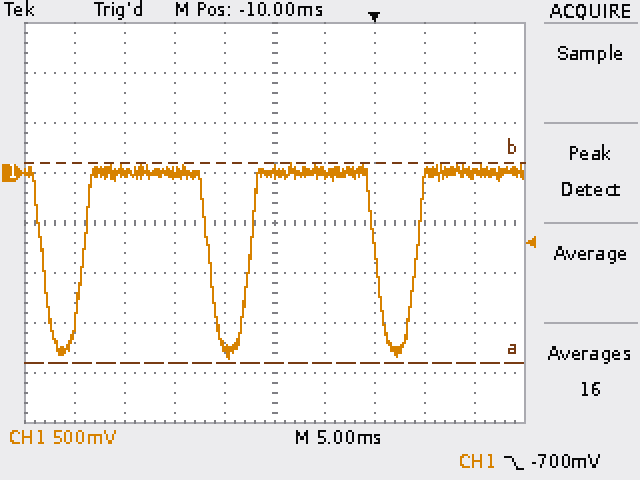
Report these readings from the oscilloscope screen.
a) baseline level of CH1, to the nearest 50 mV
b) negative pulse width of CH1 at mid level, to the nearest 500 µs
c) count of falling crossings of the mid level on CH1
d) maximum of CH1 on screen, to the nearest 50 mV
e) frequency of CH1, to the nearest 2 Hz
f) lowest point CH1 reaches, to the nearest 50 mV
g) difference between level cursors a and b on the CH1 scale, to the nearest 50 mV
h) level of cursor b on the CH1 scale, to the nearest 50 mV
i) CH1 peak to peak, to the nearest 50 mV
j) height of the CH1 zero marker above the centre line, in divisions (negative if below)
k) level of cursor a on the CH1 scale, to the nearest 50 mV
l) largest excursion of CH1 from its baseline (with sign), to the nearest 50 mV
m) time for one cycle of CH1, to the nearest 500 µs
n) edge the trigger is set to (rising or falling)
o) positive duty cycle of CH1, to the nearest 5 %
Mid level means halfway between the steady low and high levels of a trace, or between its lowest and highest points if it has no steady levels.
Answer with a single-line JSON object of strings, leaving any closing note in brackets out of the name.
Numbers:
{"baseline level of CH1, to the nearest 50 mV": "0 mV", "negative pulse width of CH1 at mid level, to the nearest 500 µs": "4.0 ms", "count of falling crossings of the mid level on CH1": "3", "maximum of CH1 on screen, to the nearest 50 mV": "100 mV", "frequency of CH1, to the nearest 2 Hz": "60 Hz", "lowest point CH1 reaches, to the nearest 50 mV": "-1.85 V", "difference between level cursors a and b on the CH1 scale, to the nearest 50 mV": "2.00 V", "level of cursor b on the CH1 scale, to the nearest 50 mV": "100 mV", "CH1 peak to peak, to the nearest 50 mV": "1.95 V", "height of the CH1 zero marker above the centre line, in divisions": "+1.0 div", "level of cursor a on the CH1 scale, to the nearest 50 mV": "-1.90 V", "largest excursion of CH1 from its baseline (with sign), to the nearest 50 mV": "-1.85 V", "time for one cycle of CH1, to the nearest 500 µs": "16.5 ms", "edge the trigger is set to": "falling", "positive duty cycle of CH1, to the nearest 5 %": "75 %"}
